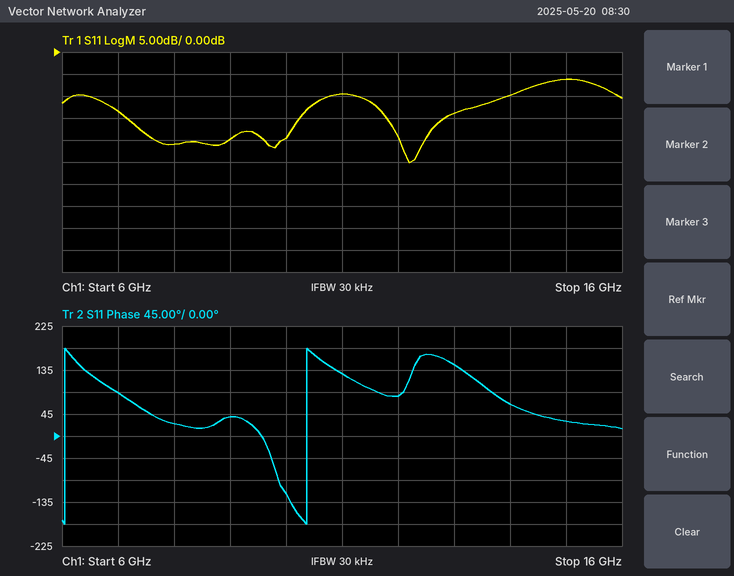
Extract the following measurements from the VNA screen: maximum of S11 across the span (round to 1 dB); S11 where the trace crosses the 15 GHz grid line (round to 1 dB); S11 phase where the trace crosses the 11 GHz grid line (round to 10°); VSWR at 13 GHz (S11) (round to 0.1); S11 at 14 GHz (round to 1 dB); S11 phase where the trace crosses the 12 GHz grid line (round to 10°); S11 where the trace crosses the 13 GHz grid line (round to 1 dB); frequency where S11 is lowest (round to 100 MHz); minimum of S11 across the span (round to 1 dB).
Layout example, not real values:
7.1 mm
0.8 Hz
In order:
-6 dB
-6 dB
130°
1.5
-10 dB
80°
-14 dB
12.2 GHz
-25 dB
